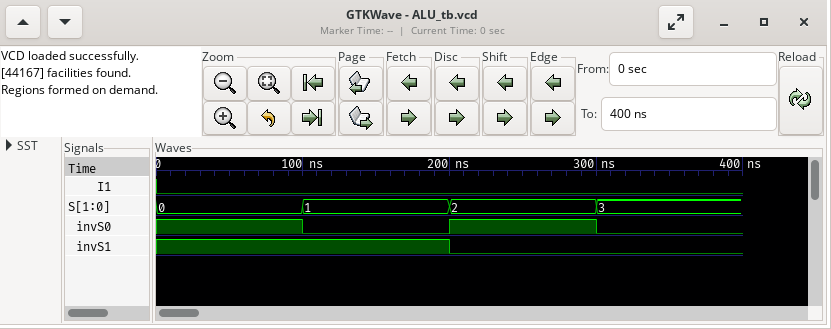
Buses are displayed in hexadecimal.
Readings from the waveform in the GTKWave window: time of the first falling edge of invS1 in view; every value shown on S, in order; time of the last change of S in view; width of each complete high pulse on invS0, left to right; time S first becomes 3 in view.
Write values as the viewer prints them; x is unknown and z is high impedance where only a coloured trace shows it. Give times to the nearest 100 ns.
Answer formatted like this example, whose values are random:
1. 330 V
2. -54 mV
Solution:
1. 200 ns
2. 0, 1, 2, 3
3. 300 ns
4. 100 ns
5. 300 ns
